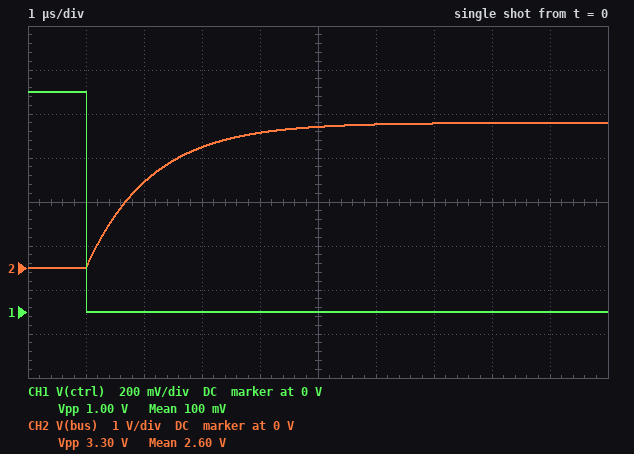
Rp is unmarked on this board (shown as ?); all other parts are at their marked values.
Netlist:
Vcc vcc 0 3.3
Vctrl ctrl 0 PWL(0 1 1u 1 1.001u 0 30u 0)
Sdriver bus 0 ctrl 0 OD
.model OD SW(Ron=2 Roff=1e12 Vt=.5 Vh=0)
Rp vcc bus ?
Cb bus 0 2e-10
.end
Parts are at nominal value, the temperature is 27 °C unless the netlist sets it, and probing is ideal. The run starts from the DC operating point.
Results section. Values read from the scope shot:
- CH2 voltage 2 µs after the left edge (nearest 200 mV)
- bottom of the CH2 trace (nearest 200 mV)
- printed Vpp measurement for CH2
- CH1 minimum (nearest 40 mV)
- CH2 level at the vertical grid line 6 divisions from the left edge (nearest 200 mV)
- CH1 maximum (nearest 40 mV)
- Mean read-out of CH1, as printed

2.0 V
0 V
3.30 V
0 V
3.2 V
1.00 V
100 mV
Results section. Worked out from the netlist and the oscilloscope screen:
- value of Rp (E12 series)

5.6 kΩ
